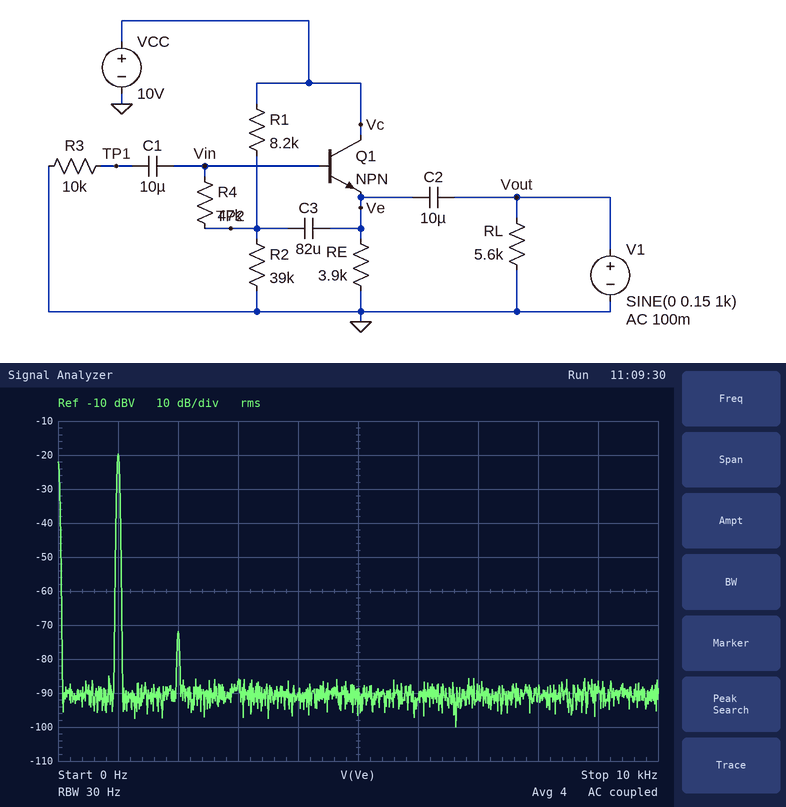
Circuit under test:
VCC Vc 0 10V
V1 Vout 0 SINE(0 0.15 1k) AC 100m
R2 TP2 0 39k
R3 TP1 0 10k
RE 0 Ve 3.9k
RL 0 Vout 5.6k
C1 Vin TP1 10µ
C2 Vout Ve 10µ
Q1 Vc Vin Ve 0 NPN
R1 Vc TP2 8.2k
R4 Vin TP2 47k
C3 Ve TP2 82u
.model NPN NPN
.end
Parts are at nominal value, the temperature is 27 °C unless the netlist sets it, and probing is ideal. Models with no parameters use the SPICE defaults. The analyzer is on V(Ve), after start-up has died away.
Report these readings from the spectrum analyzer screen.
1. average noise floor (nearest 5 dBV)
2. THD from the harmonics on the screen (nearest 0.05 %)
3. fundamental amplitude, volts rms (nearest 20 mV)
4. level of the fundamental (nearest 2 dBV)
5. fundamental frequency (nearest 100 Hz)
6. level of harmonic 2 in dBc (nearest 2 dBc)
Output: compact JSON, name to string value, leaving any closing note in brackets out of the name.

{"average noise floor": "-90 dBV", "THD from the harmonics on the screen": "0.25 %", "fundamental amplitude, volts rms": "100 mV", "level of the fundamental": "-20 dBV", "fundamental frequency": "1.0 kHz", "level of harmonic 2 in dBc": "-52 dBc"}
